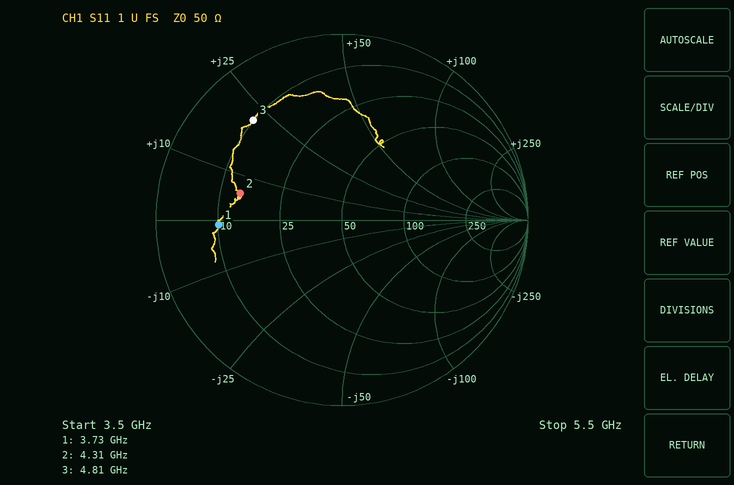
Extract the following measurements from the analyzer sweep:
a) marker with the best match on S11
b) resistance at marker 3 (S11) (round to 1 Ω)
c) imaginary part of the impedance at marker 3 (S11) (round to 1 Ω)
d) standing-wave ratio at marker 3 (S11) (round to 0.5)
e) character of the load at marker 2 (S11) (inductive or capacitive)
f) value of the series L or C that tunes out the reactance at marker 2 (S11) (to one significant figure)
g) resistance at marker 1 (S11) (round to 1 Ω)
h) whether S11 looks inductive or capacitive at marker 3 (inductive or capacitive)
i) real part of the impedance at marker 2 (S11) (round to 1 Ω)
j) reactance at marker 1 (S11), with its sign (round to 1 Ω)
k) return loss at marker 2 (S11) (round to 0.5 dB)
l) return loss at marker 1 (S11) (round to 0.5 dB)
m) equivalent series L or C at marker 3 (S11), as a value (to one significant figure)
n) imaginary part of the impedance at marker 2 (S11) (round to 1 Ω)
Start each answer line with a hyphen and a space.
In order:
- marker 2
- 10 Ω
- +22 Ω
- 6.0
- inductive
- 6 pF
- 10 Ω
- inductive
- 14 Ω
- -1 Ω
- 5.0 dB
- 3.5 dB
- 700 pH
- +6 Ω
